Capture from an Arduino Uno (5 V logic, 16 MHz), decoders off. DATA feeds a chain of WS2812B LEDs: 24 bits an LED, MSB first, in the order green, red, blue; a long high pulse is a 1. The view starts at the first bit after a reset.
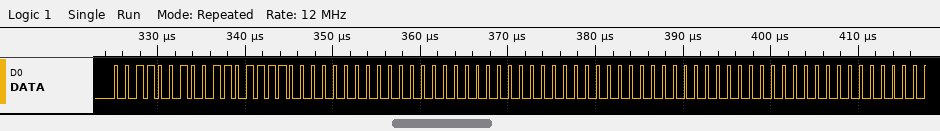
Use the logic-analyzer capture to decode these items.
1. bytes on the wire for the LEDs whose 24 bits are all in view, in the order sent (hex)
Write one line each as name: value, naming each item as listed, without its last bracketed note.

bytes on the wire for the LEDs whose 24 bits are all in view, in the order sent: 32 6F 00 00 00 00 00 00 00
